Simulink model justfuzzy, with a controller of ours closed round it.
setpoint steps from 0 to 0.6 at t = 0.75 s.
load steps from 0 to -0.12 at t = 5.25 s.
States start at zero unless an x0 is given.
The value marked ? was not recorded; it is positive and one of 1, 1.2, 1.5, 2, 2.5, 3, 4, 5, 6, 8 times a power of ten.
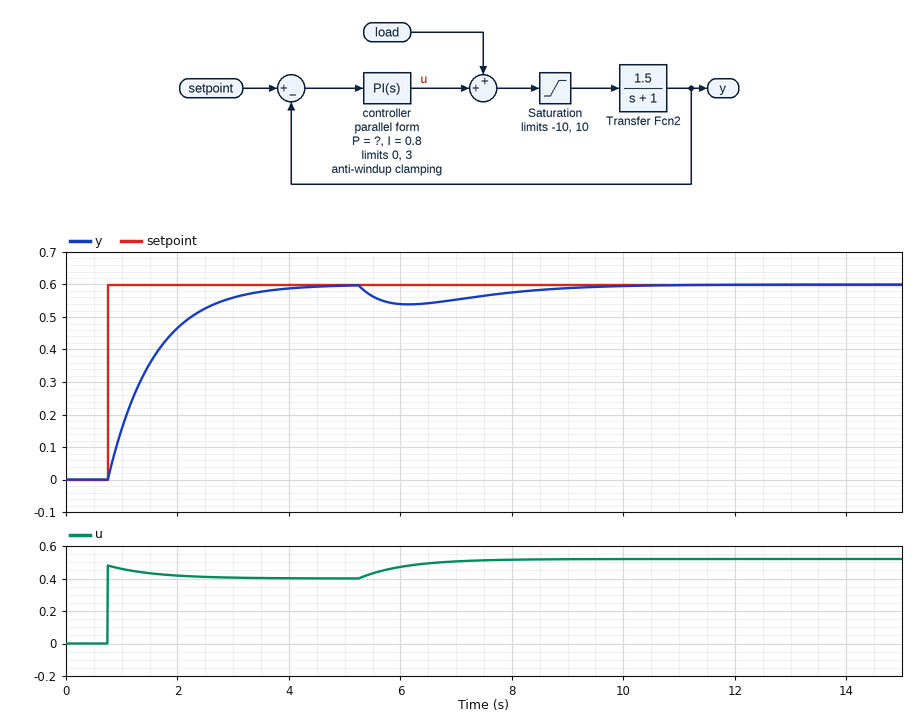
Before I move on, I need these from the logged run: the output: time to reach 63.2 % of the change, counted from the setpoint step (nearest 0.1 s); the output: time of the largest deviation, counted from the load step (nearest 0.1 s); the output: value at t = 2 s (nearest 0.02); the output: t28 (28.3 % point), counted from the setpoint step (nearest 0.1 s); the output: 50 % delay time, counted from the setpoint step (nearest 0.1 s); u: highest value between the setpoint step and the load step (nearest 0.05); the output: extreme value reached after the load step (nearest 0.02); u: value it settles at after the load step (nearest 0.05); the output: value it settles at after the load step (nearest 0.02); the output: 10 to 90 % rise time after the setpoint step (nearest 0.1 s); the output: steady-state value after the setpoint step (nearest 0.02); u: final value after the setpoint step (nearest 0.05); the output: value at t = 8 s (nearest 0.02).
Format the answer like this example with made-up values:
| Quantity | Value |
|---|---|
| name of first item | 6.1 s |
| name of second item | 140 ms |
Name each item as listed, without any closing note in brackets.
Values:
| Quantity | Value |
|---|---|
| the output: time to reach 63.2 % of the change, counted from the setpoint step | 0.8 s |
| the output: time of the largest deviation, counted from the load step | 0.9 s |
| the output: value at t = 2 s | 0.46 |
| the output: t28 (28.3 % point), counted from the setpoint step | 0.3 s |
| the output: 50 % delay time, counted from the setpoint step | 0.6 s |
| u: highest value between the setpoint step and the load step | 0.50 |
| the output: extreme value reached after the load step | 0.54 |
| u: value it settles at after the load step | 0.50 |
| the output: value it settles at after the load step | 0.60 |
| the output: 10 to 90 % rise time after the setpoint step | 1.8 s |
| the output: steady-state value after the setpoint step | 0.60 |
| u: final value after the setpoint step | 0.40 |
| the output: value at t = 8 s | 0.58 |
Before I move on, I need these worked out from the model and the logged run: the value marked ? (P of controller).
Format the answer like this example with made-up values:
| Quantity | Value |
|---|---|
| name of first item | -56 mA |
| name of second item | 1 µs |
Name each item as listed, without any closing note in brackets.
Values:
| Quantity | Value |
|---|---|
| the value marked ? | 0.8 |
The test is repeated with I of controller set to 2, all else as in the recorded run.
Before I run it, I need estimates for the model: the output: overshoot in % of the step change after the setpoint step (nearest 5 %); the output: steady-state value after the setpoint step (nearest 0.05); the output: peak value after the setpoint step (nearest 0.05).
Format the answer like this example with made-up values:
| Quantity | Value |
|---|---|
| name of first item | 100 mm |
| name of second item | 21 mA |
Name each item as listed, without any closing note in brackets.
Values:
| Quantity | Value |
|---|---|
| the output: overshoot in % of the step change after the setpoint step | 10 % |
| the output: steady-state value after the setpoint step | 0.60 |
| the output: peak value after the setpoint step | 0.65 |
